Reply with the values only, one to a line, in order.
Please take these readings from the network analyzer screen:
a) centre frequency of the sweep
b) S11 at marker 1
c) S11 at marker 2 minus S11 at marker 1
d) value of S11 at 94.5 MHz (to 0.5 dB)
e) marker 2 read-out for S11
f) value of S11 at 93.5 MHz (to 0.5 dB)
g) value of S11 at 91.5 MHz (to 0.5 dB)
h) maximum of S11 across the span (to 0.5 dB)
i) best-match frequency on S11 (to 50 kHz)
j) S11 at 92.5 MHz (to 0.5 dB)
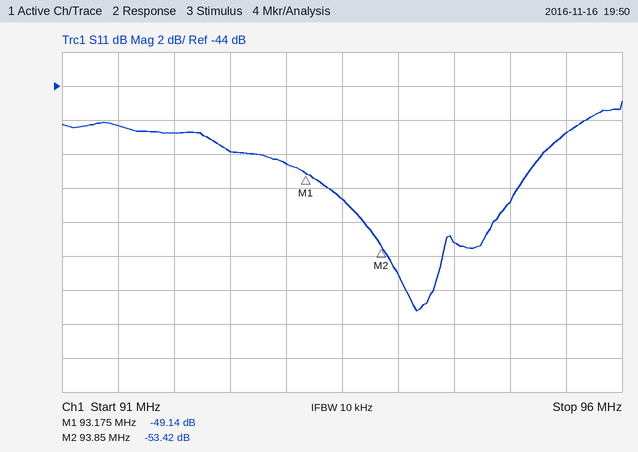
93.5 MHz
-49.14 dB
-4.28 dB
-53.0 dB
-53.42 dB
-50.5 dB
-46.5 dB
-45.0 dB
94.15 MHz
-48.0 dB
